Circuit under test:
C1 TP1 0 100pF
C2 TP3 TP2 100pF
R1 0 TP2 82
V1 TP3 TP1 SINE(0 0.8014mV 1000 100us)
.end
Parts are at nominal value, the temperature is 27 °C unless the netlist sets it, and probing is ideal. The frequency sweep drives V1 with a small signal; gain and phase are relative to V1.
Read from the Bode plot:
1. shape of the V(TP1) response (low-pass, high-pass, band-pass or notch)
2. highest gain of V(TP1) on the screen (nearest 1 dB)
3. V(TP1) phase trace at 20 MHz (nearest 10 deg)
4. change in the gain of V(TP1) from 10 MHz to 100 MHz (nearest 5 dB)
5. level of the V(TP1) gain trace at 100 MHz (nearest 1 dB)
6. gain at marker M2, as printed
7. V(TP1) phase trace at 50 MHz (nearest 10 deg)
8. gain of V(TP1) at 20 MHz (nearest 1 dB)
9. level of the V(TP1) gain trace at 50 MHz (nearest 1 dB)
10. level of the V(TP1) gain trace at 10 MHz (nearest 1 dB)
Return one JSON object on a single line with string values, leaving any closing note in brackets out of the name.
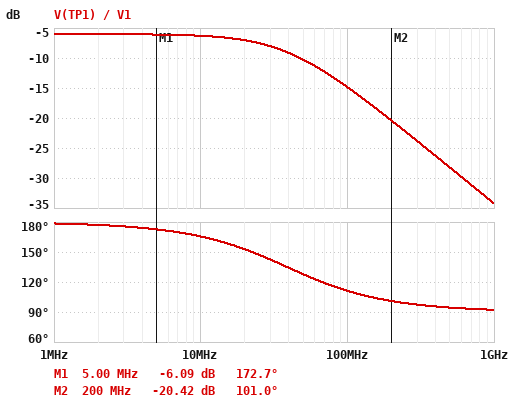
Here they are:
{"shape of the V(TP1) response": "low-pass", "highest gain of V(TP1) on the screen": "-6 dB", "V(TP1) phase trace at 20 MHz": "150 deg", "change in the gain of V(TP1) from 10 MHz to 100 MHz": "-10 dB", "level of the V(TP1) gain trace at 100 MHz": "-15 dB", "gain at marker M2, as printed": "-20.42 dB", "V(TP1) phase trace at 50 MHz": "130 deg", "gain of V(TP1) at 20 MHz": "-7 dB", "level of the V(TP1) gain trace at 50 MHz": "-10 dB", "level of the V(TP1) gain trace at 10 MHz": "-6 dB"}
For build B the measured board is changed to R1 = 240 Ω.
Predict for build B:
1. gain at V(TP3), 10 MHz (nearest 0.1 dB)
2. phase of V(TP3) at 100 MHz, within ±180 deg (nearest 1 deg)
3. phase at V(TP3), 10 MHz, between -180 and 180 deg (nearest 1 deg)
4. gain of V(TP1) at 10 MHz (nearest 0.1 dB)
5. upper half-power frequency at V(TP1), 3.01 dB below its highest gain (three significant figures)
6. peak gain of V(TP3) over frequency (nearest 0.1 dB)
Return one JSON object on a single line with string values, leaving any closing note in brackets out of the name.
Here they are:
{"gain at V(TP3), 10 MHz": "-2.8 dB", "phase of V(TP3) at 100 MHz, within ±180 deg": "4 deg", "phase at V(TP3), 10 MHz, between -180 and 180 deg": "19 deg", "gain of V(TP1) at 10 MHz": "-8.0 dB", "upper half-power frequency at V(TP1), 3.01 dB below its highest gain": "13.3 MHz", "peak gain of V(TP3) over frequency": "0 dB"}
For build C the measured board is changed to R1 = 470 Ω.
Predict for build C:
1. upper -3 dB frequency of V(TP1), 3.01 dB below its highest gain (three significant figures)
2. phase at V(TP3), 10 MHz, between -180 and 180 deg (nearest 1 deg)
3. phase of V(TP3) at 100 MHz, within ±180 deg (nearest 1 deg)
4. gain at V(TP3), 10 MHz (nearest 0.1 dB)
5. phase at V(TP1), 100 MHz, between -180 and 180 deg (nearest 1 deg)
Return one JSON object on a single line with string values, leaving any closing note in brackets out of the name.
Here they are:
{"upper -3 dB frequency of V(TP1), 3.01 dB below its highest gain": "6.77 MHz", "phase at V(TP3), 10 MHz, between -180 and 180 deg": "15 deg", "phase of V(TP3) at 100 MHz, within ±180 deg": "2 deg", "gain at V(TP3), 10 MHz": "-1.2 dB", "phase at V(TP1), 100 MHz, between -180 and 180 deg": "94 deg"}
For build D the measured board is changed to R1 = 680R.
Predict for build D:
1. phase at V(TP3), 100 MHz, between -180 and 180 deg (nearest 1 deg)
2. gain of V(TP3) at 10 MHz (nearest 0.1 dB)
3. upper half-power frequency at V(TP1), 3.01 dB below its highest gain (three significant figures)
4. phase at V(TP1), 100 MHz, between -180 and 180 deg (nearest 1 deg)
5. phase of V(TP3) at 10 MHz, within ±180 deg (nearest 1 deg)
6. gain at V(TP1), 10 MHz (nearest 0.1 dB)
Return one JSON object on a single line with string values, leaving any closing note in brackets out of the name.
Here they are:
{"phase at V(TP3), 100 MHz, between -180 and 180 deg": "1 deg", "gain of V(TP3) at 10 MHz": "-0.6 dB", "upper half-power frequency at V(TP1), 3.01 dB below its highest gain": "4.68 MHz", "phase at V(TP1), 100 MHz, between -180 and 180 deg": "93 deg", "phase of V(TP3) at 10 MHz, within ±180 deg": "12 deg", "gain at V(TP1), 10 MHz": "-13.5 dB"}
